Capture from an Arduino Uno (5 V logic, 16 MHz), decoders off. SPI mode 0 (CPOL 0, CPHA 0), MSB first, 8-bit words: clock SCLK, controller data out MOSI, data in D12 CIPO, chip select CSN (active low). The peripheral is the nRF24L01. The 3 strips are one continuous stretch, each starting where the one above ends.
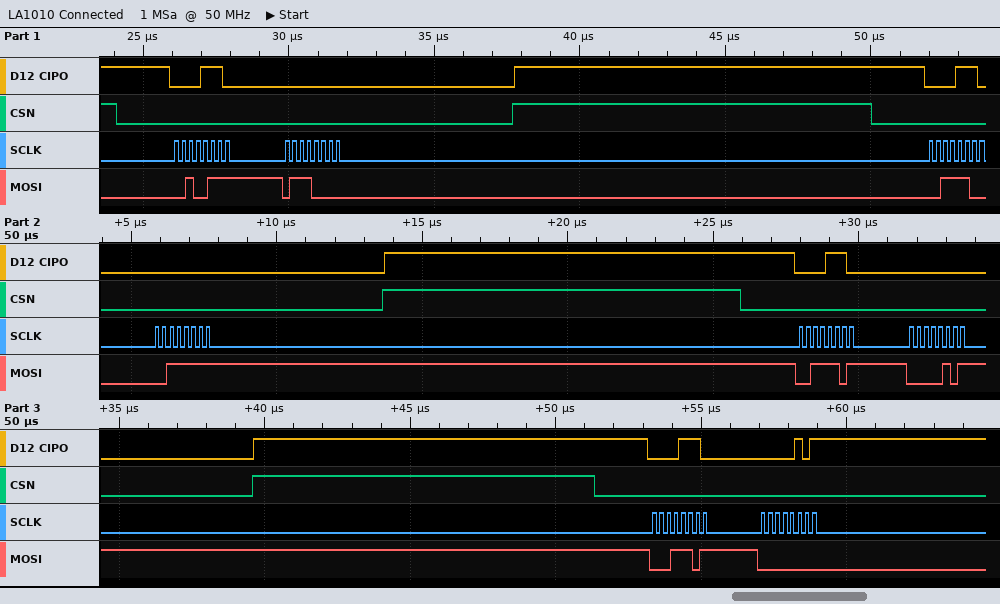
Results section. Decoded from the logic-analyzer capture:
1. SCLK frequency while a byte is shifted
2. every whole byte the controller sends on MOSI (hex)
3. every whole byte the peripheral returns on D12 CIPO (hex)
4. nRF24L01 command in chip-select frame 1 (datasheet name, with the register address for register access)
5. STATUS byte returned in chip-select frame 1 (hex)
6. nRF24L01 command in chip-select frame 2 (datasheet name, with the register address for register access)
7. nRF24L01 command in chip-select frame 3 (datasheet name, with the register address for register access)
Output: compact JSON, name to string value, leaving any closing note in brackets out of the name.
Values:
{"SCLK frequency while a byte is shifted": "4 MHz", "every whole byte the controller sends on MOSI": "27 70 3C 3F 3D 05 1D 00", "every whole byte the peripheral returns on D12 CIPO": "0E 00 0E 00 0E 00 0E 05", "nRF24L01 command in chip-select frame 1": "W_REGISTER 0x07", "STATUS byte returned in chip-select frame 1": "0x0E", "nRF24L01 command in chip-select frame 2": "W_REGISTER 0x1C", "nRF24L01 command in chip-select frame 3": "W_REGISTER 0x1D"}
